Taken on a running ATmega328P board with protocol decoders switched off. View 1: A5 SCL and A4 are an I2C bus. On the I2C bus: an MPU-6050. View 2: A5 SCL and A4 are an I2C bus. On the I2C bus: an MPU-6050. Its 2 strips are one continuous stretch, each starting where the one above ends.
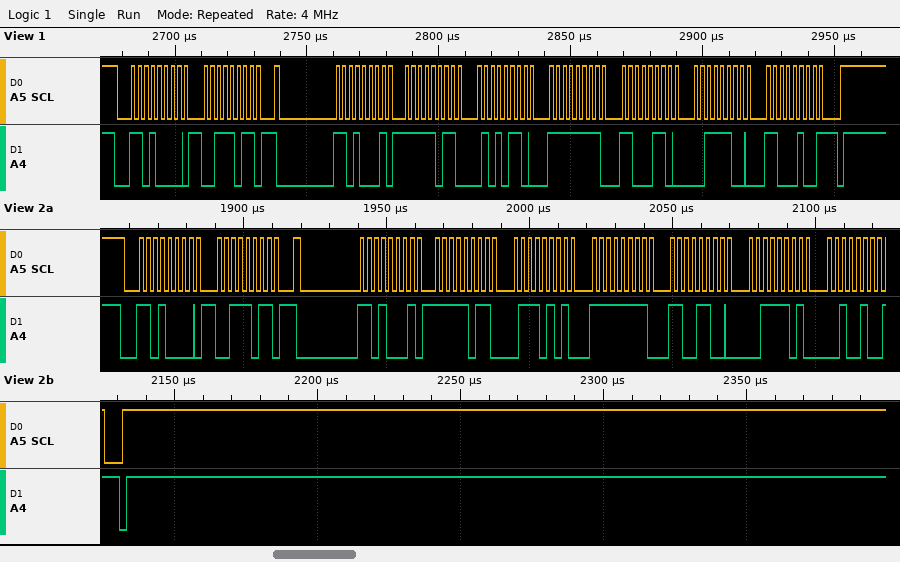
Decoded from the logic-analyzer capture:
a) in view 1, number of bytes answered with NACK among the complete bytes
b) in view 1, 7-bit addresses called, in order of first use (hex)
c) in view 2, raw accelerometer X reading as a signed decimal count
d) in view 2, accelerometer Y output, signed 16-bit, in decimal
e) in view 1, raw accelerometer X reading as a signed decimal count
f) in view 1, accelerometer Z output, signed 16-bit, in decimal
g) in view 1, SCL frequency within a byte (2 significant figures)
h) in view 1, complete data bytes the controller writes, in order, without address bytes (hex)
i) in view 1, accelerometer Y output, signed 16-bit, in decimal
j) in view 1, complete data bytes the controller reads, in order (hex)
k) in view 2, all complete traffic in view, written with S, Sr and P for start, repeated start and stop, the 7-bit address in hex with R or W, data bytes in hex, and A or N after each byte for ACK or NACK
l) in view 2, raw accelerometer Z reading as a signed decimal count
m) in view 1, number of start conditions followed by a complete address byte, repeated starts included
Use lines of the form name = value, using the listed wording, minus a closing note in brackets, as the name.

in view 1, number of bytes answered with NACK among the complete bytes = 1
in view 1, 7-bit addresses called, in order of first use = 0x68
in view 2, raw accelerometer X reading as a signed decimal count = -1163
in view 2, accelerometer Y output, signed 16-bit, in decimal = -52
in view 1, raw accelerometer X reading as a signed decimal count = -1194
in view 1, accelerometer Z output, signed 16-bit, in decimal = 15556
in view 1, SCL frequency within a byte = 400 kHz
in view 1, complete data bytes the controller writes, in order, without address bytes = 3B
in view 1, accelerometer Y output, signed 16-bit, in decimal = -58
in view 1, complete data bytes the controller reads, in order = FB 56 FF C6 3C C4
in view 2, all complete traffic in view, written with S, Sr and P for start, repeated start and stop, the 7-bit address in hex with R or W, data bytes in hex, and A or N after each byte for ACK or NACK = S 68W A 3B A Sr 68R A FB A 75 A FF A CC A 3D A 24 N P
in view 2, raw accelerometer Z reading as a signed decimal count = 15652
in view 1, number of start conditions followed by a complete address byte, repeated starts included = 2
